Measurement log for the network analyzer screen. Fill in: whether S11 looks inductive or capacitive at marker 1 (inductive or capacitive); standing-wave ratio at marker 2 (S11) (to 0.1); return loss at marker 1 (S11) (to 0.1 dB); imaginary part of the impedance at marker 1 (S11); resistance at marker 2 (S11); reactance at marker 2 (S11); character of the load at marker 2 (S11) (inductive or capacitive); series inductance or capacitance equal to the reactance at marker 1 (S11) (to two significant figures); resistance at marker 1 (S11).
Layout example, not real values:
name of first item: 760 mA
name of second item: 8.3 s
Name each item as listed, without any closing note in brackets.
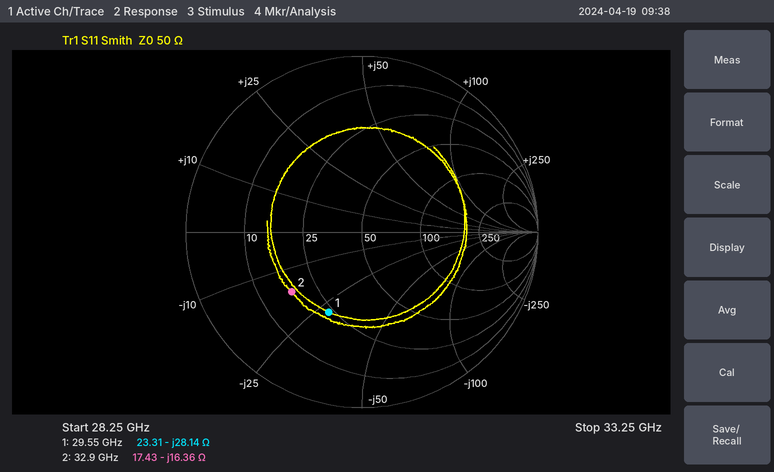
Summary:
whether S11 looks inductive or capacitive at marker 1: capacitive
standing-wave ratio at marker 2 (S11): 3.2
return loss at marker 1 (S11): 6.1 dB
imaginary part of the impedance at marker 1: -28.14 Ω
resistance at marker 2: 17.43 Ω
reactance at marker 2: -16.36 Ω
character of the load at marker 2 (S11): capacitive
series inductance or capacitance equal to the reactance at marker 1 (S11): 190 fF
resistance at marker 1: 23.31 Ω
